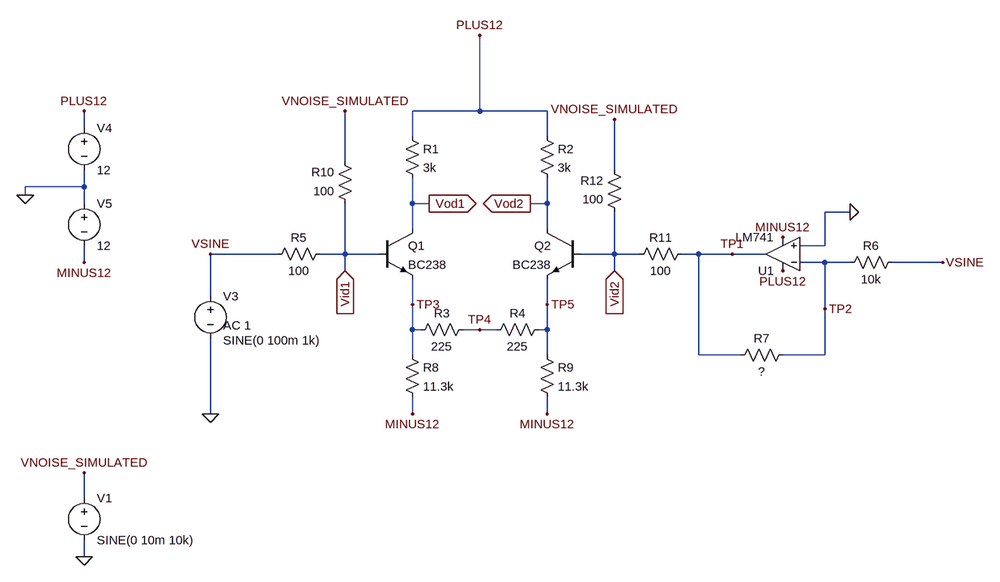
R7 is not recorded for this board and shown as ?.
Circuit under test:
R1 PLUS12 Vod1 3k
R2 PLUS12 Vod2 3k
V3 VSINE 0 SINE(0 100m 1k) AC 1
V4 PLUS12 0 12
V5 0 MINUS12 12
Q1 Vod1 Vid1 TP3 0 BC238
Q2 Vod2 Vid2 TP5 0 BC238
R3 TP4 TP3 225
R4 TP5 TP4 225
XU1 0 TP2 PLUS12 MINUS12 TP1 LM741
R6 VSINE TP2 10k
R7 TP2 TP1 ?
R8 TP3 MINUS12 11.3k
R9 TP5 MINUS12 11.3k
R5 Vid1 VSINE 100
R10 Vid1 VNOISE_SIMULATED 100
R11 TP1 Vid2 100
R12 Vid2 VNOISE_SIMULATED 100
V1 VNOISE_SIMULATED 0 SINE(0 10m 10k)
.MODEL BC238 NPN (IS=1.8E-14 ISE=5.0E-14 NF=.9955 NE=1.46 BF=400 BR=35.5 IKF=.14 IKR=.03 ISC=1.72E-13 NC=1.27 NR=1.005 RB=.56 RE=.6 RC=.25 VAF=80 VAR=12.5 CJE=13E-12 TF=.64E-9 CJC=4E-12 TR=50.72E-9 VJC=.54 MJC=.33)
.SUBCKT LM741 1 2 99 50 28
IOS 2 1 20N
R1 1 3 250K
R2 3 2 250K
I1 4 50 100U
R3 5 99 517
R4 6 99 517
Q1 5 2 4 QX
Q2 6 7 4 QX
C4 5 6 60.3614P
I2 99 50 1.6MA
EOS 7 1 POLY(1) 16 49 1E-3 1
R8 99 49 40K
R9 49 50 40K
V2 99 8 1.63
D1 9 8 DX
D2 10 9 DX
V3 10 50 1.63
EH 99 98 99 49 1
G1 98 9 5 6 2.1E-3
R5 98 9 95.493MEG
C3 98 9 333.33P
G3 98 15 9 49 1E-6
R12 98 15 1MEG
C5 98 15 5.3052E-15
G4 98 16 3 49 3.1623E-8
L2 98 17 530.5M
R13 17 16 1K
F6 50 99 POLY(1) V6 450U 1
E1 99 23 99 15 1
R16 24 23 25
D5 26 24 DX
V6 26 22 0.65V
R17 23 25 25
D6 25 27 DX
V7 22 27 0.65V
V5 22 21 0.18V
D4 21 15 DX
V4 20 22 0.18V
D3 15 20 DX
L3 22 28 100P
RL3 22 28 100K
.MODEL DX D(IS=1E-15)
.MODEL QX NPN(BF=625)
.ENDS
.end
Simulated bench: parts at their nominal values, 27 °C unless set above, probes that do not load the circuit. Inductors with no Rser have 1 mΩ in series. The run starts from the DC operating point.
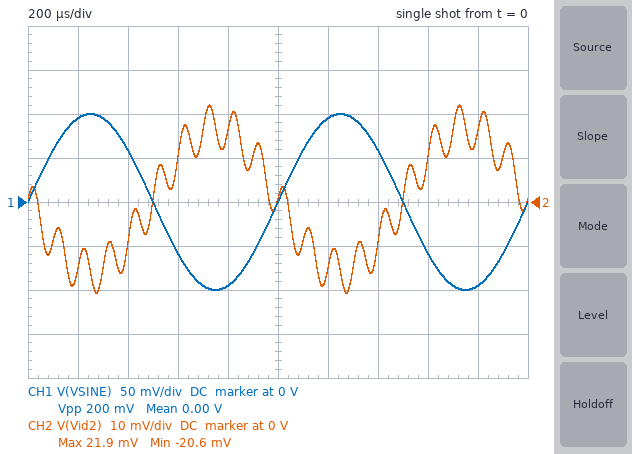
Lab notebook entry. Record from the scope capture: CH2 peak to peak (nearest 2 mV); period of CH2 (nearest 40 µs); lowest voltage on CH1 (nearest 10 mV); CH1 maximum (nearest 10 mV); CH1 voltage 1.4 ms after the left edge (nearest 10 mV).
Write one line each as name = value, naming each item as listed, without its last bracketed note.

CH2 peak to peak = 42 mV
period of CH2 = 1.00 ms
lowest voltage on CH1 = -100 mV
CH1 maximum = 100 mV
CH1 voltage 1.4 ms after the left edge = 60 mV
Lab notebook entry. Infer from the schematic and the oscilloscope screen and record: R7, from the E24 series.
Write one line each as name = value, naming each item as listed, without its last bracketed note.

R7, from the E24 series = 3.3 kΩ
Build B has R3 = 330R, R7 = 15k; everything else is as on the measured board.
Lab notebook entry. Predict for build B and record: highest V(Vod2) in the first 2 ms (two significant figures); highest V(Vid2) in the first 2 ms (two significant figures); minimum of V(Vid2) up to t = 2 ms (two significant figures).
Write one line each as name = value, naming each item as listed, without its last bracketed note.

highest V(Vod2) in the first 2 ms = 9.6 V
highest V(Vid2) in the first 2 ms = 81 mV
minimum of V(Vid2) up to t = 2 ms = -77 mV
